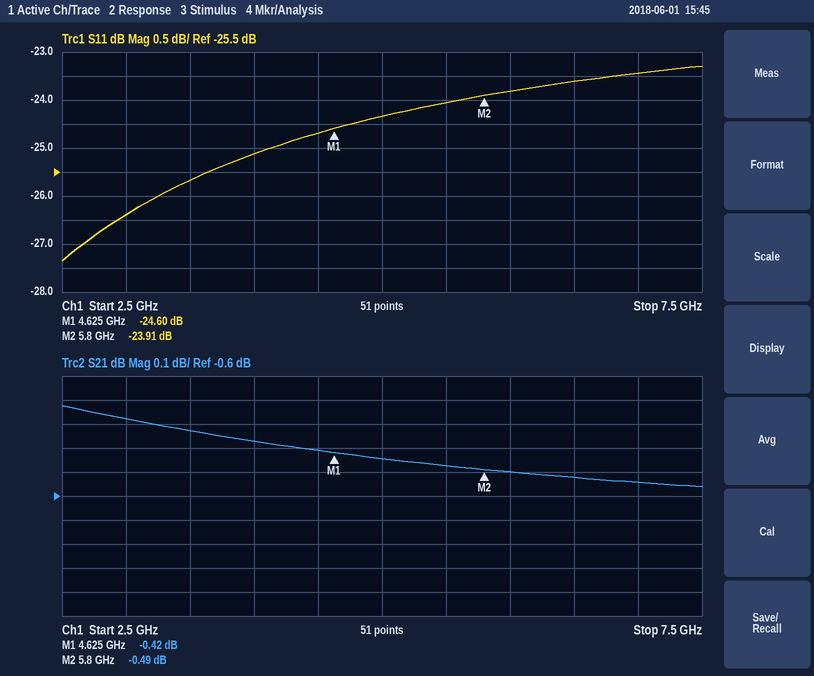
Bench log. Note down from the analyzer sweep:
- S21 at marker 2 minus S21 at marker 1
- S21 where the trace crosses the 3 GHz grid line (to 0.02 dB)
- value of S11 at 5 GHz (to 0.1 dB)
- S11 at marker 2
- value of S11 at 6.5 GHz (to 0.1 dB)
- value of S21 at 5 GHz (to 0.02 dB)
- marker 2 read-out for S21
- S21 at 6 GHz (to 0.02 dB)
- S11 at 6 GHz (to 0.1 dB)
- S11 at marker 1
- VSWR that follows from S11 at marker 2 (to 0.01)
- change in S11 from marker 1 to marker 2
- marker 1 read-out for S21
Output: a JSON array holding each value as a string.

["-0.07 dB", "-0.28 dB", "-24.3 dB", "-23.91 dB", "-23.6 dB", "-0.44 dB", "-0.49 dB", "-0.50 dB", "-23.8 dB", "-24.60 dB", "1.14", "0.69 dB", "-0.42 dB"]
